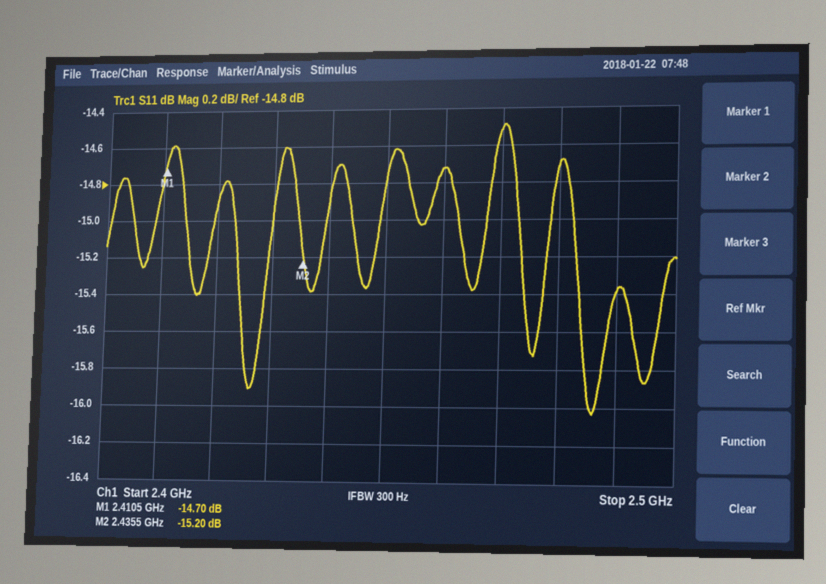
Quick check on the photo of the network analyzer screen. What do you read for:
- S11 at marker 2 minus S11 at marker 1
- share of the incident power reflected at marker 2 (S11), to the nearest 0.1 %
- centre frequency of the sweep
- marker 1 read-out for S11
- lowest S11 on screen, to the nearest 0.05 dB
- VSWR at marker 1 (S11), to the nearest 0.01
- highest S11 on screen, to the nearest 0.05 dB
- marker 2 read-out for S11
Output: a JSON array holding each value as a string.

["-0.50 dB", "3.0 %", "2.45 GHz", "-14.70 dB", "-16.05 dB", "1.45", "-14.50 dB", "-15.20 dB"]
